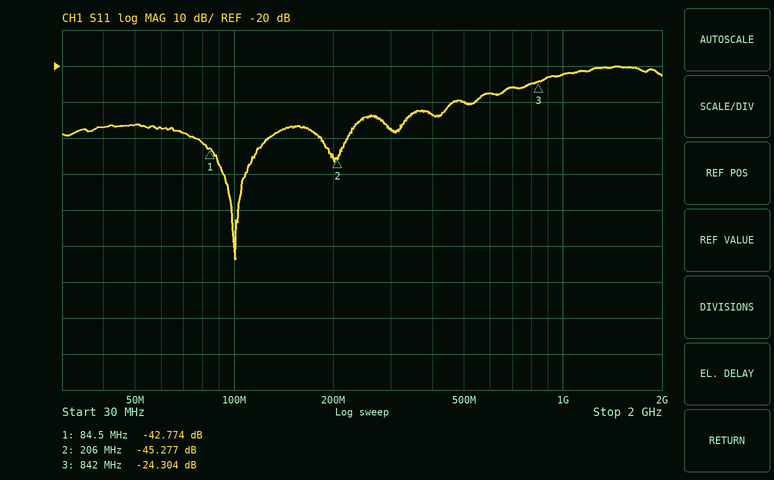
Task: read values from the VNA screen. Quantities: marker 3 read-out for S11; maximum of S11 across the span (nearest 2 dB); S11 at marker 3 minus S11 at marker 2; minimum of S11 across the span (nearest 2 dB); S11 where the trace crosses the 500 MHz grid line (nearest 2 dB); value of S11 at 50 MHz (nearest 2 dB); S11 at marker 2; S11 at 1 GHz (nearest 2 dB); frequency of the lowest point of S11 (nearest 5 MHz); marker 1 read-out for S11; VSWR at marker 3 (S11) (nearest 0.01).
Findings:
-24.304 dB
-20 dB
20.973 dB
-74 dB
-30 dB
-36 dB
-45.277 dB
-22 dB
100 MHz
-42.774 dB
1.13
